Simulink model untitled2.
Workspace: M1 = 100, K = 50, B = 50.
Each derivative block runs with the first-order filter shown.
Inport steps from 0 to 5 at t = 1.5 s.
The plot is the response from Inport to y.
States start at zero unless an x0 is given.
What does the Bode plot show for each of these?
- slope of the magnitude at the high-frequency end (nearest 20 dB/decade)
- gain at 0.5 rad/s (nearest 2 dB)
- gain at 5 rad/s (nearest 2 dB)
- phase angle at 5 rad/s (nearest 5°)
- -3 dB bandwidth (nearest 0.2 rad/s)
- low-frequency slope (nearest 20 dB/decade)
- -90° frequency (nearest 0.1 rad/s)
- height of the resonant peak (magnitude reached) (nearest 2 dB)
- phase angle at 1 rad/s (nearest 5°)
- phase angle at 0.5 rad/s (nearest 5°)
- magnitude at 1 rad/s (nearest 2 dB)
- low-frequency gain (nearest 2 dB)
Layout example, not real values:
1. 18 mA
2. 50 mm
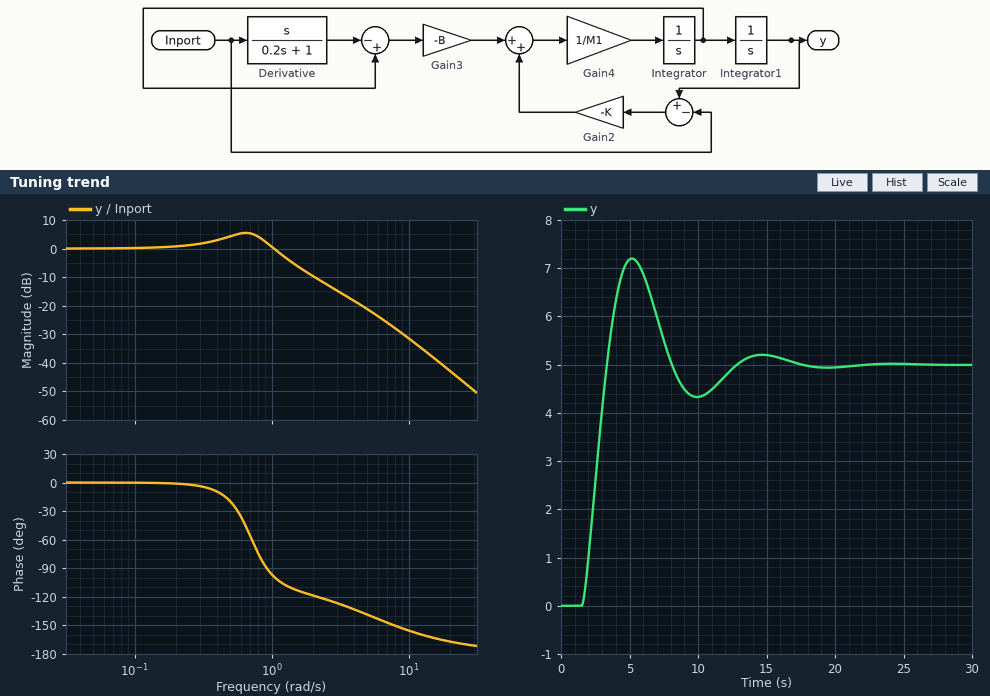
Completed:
1. -40 dB/decade
2. 4 dB
3. -22 dB
4. -140°
5. 1.2 rad/s
6. 0 dB/decade
7. 0.9 rad/s
8. 6 dB
9. -95°
10. -20°
11. 0 dB
12. 0 dB
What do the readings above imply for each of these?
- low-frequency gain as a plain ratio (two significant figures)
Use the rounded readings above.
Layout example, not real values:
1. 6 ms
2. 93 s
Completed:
1. 1.0
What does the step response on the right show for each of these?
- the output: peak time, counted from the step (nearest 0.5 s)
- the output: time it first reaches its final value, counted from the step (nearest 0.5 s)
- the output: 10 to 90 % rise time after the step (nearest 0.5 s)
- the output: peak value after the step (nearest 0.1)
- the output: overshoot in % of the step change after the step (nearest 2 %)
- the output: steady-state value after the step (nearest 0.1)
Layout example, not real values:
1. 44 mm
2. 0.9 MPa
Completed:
1. 3.5 s
2. 2.0 s
3. 1.5 s
4. 7.2
5. 44 %
6. 5.0
